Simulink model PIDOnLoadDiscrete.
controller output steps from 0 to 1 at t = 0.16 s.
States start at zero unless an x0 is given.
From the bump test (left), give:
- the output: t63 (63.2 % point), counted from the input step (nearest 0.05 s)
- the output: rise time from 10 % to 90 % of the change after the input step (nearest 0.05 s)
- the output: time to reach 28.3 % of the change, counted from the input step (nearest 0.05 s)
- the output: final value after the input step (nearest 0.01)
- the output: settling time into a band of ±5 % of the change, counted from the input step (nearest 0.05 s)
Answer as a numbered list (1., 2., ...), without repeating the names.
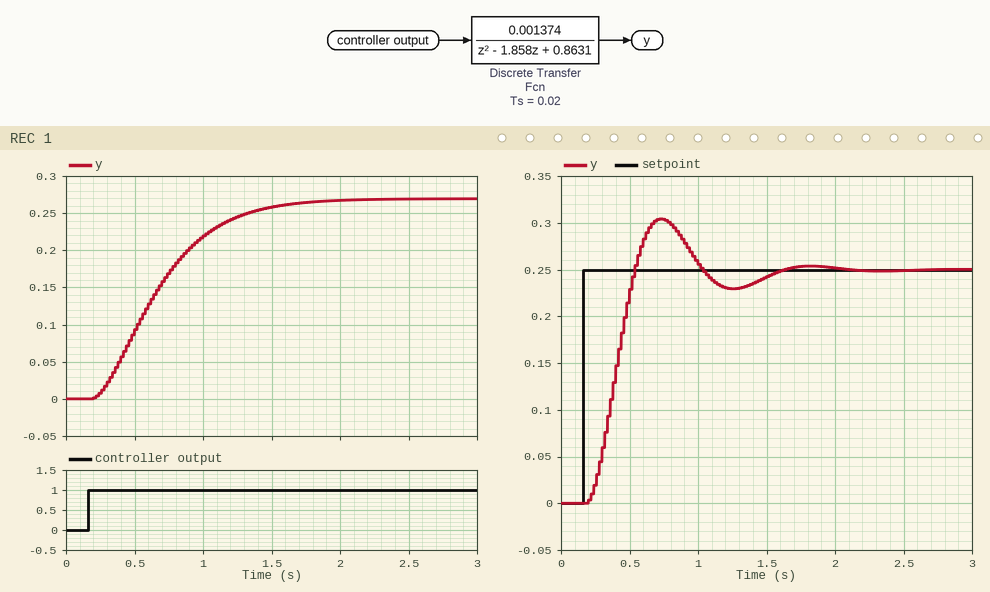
1. 0.60 s
2. 0.90 s
3. 0.30 s
4. 0.27
5. 1.30 s
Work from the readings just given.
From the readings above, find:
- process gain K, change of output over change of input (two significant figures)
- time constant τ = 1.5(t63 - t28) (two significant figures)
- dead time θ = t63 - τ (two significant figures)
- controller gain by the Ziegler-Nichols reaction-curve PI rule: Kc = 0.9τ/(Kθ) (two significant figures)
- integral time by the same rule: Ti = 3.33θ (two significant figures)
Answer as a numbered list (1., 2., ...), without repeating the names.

1. 0.27
2. 0.45 s
3. 0.15 s
4. 10
5. 0.50 s
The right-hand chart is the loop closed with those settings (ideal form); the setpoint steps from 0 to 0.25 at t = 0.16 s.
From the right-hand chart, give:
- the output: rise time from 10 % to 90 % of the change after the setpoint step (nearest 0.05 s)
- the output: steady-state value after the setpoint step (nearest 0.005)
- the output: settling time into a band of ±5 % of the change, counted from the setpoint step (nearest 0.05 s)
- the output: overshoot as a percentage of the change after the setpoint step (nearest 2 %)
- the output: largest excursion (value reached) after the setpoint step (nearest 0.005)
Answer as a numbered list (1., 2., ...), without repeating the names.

1. 0.25 s
2. 0.250
3. 1.30 s
4. 22 %
5. 0.305
